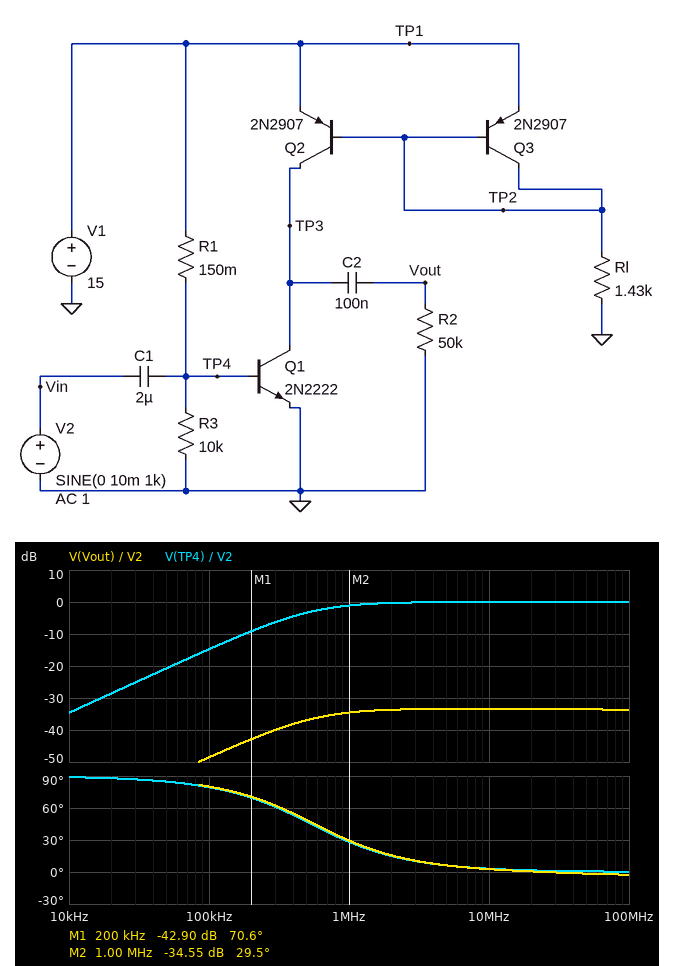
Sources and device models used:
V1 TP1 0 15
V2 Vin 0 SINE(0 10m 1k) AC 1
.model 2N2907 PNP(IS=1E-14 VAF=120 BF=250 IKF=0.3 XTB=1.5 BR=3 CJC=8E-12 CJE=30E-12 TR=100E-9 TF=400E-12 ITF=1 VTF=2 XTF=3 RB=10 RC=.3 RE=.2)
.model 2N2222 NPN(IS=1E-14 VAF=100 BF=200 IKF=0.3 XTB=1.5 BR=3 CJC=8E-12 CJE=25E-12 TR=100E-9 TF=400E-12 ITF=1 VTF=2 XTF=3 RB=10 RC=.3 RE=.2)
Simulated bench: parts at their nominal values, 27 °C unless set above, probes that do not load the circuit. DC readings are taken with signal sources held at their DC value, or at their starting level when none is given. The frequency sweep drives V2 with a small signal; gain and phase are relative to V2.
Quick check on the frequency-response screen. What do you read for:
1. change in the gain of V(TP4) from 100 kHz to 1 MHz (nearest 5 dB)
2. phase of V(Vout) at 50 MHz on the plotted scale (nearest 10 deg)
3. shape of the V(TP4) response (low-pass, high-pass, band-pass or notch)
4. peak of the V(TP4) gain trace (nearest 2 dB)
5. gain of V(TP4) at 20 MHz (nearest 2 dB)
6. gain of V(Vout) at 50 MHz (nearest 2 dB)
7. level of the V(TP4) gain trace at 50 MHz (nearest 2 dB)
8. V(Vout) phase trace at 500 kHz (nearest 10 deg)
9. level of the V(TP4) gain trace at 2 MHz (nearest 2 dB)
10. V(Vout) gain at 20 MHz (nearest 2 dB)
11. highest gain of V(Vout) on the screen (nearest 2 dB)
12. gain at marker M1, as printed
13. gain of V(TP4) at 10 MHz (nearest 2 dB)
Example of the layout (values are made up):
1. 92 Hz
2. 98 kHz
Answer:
1. 15 dB
2. 0 deg
3. high-pass
4. 0 dB
5. 0 dB
6. -34 dB
7. 0 dB
8. 50 deg
9. 0 dB
10. -34 dB
11. -34 dB
12. -42.90 dB
13. 0 dB
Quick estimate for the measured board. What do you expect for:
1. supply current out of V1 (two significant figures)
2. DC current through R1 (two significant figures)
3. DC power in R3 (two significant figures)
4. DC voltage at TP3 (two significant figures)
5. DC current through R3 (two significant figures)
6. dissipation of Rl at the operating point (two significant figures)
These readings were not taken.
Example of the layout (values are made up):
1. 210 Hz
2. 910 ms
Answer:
1. 1.4 A
2. 1.4 A
3. 22 mW
4. 310 mV
5. 1.5 mA
6. 140 mW
